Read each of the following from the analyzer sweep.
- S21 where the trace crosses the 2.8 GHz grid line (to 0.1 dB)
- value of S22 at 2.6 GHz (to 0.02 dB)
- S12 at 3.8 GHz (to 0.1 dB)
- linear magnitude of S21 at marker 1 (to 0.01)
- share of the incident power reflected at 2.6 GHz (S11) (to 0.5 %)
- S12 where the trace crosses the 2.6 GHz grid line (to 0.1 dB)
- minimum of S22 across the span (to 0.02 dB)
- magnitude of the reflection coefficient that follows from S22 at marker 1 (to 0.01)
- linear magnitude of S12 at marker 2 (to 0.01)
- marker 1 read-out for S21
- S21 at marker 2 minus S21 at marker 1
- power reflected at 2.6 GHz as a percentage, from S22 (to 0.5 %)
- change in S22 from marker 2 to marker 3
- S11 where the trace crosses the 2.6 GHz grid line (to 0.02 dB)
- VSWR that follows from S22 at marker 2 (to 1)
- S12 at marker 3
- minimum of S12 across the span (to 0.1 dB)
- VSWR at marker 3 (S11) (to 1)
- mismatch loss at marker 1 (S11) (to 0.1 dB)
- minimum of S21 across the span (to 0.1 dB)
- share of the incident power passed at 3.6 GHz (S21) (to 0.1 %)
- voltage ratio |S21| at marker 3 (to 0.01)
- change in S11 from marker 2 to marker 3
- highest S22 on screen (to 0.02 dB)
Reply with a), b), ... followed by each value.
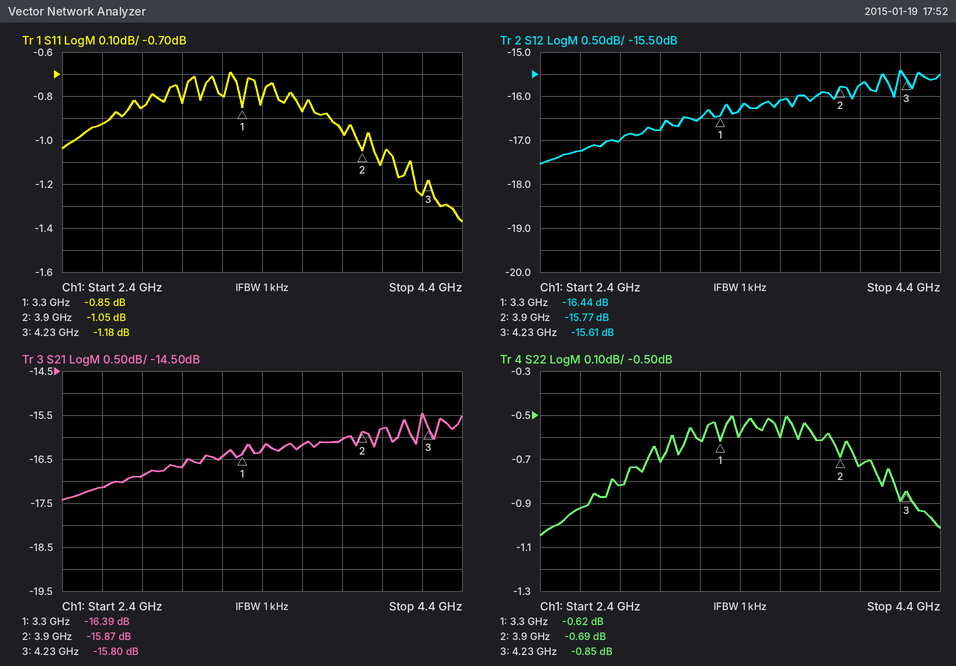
a) -16.9 dB
b) -0.92 dB
c) -15.9 dB
d) 0.15
e) 81.0 %
f) -17.2 dB
g) -1.04 dB
h) 0.93
i) 0.16
j) -16.39 dB
k) 0.52 dB
l) 81.0 %
m) -0.16 dB
n) -0.92 dB
o) 25
p) -15.61 dB
q) -17.5 dB
r) 15
s) 7.5 dB
t) -17.4 dB
u) 2.4 %
v) 0.16
w) -0.13 dB
x) -0.50 dB
